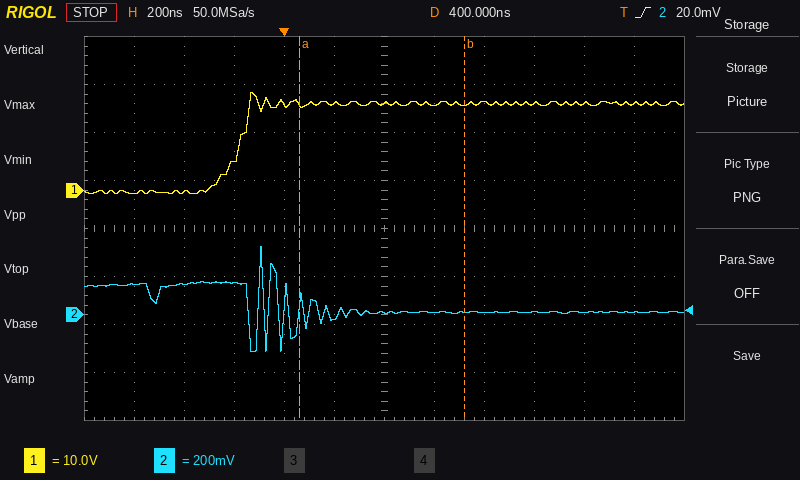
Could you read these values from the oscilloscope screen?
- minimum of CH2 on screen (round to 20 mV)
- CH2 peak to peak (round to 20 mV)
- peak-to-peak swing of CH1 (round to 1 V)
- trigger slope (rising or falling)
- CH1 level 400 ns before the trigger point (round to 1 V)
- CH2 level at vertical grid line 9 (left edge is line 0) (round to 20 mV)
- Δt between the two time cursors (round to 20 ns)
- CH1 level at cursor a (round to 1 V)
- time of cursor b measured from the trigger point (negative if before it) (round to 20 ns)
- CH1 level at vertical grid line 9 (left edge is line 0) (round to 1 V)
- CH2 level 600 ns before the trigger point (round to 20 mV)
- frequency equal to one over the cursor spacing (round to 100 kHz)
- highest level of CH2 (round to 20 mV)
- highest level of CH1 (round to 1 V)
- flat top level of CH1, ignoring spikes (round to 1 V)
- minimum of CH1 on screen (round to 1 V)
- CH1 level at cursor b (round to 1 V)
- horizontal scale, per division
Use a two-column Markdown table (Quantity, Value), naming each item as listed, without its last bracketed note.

| Quantity | Value |
|---|---|
| minimum of CH2 on screen | -160 mV |
| CH2 peak to peak | 440 mV |
| peak-to-peak swing of CH1 | 21 V |
| trigger slope | rising |
| CH1 level 400 ns before the trigger point | 0 V |
| CH2 level at vertical grid line 9 (left edge is line 0) | 20 mV |
| Δt between the two time cursors | 660 ns |
| CH1 level at cursor a | 18 V |
| time of cursor b measured from the trigger point (negative if before it) | +720 ns |
| CH1 level at vertical grid line 9 (left edge is line 0) | 18 V |
| CH2 level 600 ns before the trigger point | 120 mV |
| frequency equal to one over the cursor spacing | 1.5 MHz |
| highest level of CH2 | 280 mV |
| highest level of CH1 | 20 V |
| flat top level of CH1, ignoring spikes | 18 V |
| minimum of CH1 on screen | -1 V |
| CH1 level at cursor b | 18 V |
| horizontal scale, per division | 200 ns |
